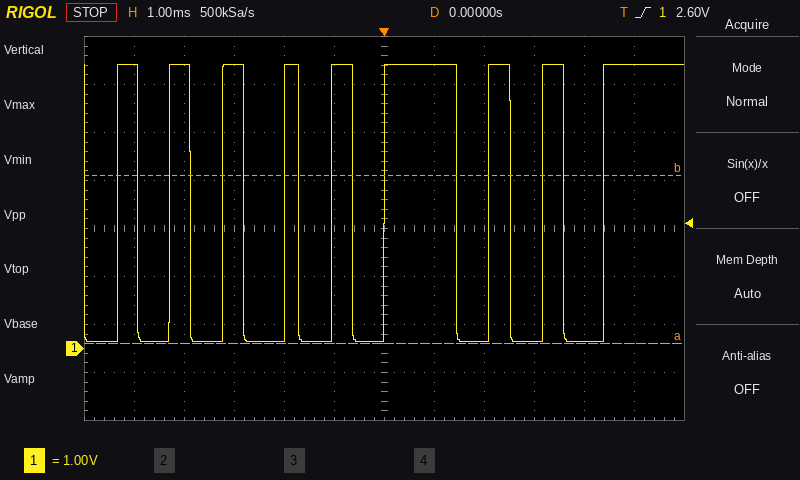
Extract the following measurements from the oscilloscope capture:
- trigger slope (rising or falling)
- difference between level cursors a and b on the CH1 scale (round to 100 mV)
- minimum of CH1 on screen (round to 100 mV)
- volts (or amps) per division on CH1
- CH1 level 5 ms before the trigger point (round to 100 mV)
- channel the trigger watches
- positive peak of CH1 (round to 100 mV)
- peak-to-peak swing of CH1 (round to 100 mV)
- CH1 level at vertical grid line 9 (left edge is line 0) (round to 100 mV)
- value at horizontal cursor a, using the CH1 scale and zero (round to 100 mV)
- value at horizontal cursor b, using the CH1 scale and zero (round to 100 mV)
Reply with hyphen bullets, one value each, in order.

- rising
- 3.5 V
- 100 mV
- 1 V
- 5.9 V
- CH1
- 5.9 V
- 5.8 V
- 100 mV
- 100 mV
- 3.6 V
